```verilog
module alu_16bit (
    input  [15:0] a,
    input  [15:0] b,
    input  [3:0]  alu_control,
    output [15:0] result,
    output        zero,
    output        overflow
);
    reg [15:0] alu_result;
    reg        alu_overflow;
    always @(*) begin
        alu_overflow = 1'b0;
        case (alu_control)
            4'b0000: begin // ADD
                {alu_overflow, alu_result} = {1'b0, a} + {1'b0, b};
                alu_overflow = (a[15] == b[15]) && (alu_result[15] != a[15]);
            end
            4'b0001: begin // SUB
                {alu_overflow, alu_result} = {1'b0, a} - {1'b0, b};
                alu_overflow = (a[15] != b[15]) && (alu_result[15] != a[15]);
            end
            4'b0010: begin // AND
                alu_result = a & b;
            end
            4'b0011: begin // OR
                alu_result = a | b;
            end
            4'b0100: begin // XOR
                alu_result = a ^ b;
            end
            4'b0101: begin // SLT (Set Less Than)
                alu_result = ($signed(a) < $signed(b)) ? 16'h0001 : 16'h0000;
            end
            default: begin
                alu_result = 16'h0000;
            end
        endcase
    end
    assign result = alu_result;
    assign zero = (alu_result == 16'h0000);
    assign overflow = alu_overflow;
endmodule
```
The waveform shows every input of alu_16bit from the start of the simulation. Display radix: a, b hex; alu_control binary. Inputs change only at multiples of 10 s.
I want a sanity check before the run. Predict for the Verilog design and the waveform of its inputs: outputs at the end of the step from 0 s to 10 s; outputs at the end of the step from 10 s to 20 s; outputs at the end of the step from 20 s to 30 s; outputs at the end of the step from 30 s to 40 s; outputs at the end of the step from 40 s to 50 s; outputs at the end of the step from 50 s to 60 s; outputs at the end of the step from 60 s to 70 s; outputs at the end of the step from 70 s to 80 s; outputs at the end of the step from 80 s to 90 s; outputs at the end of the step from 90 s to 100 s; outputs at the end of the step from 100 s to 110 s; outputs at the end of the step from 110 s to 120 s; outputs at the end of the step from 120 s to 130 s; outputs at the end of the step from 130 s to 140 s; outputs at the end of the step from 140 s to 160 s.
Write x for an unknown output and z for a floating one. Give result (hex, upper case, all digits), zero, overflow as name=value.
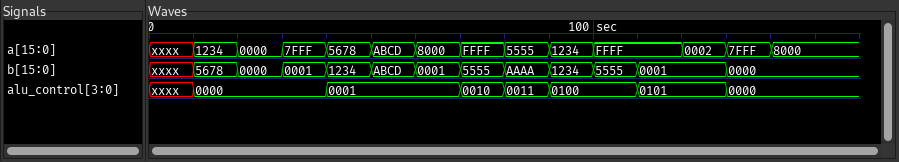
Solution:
result=x, zero=x, overflow=x
result=68AC, zero=0, overflow=0
result=0000, zero=1, overflow=0
result=8000, zero=0, overflow=1
result=4444, zero=0, overflow=0
result=0000, zero=1, overflow=0
result=7FFF, zero=0, overflow=1
result=5555, zero=0, overflow=0
result=FFFF, zero=0, overflow=0
result=0000, zero=1, overflow=0
result=AAAA, zero=0, overflow=0
result=0001, zero=0, overflow=0
result=0000, zero=1, overflow=0
result=7FFF, zero=0, overflow=0
result=8000, zero=0, overflow=0
